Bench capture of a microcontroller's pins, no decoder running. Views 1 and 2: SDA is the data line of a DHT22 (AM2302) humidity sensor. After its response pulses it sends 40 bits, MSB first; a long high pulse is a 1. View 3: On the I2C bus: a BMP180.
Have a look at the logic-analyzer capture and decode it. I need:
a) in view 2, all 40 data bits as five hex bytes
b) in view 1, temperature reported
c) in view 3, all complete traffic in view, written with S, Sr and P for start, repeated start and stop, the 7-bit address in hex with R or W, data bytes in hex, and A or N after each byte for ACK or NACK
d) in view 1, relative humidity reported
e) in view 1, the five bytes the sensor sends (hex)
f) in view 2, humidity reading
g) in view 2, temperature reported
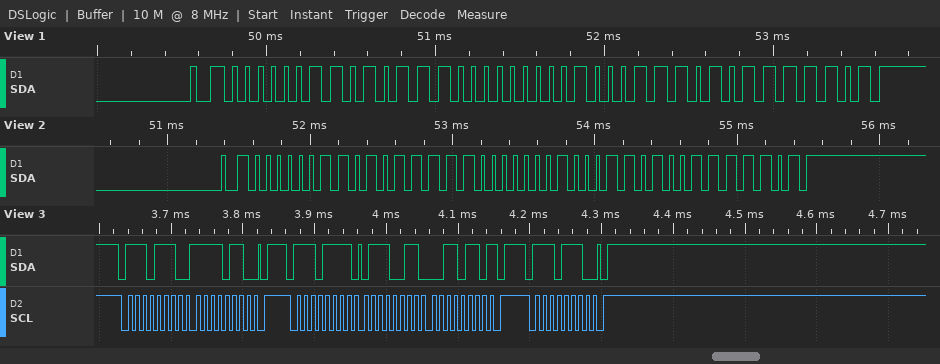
03 5F 01 1A 7D
28.5 °C
S 77W A F6 A P S 77R A 73 A 36 N P S 77W A P
86.0 %
03 5C 01 1D 7D
86.3 %
28.2 °C
